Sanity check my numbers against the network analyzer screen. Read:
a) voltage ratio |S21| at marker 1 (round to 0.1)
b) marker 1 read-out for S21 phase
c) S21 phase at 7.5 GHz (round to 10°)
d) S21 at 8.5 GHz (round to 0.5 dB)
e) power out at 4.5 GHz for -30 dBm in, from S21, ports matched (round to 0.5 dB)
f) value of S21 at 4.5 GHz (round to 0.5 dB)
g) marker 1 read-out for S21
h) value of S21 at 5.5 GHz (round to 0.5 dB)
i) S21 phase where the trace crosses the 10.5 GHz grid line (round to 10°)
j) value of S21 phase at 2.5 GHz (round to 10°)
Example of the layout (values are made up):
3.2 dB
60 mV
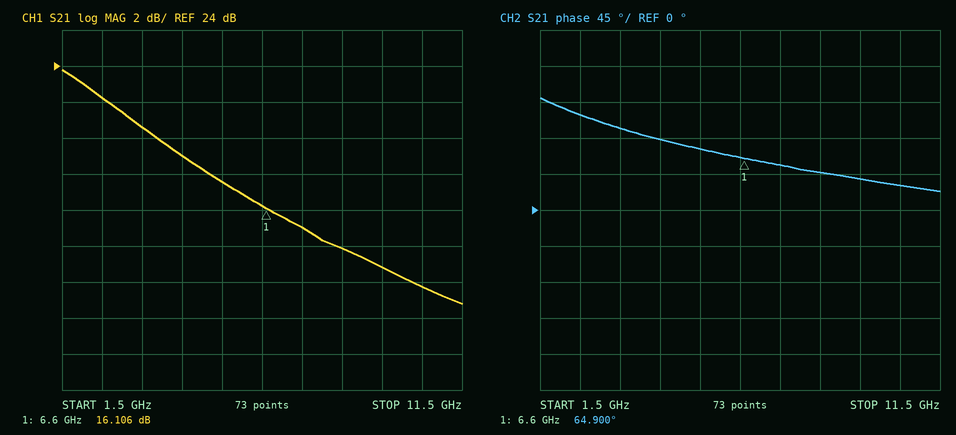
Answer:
6.4
64.900°
60°
14.0 dB
-11.0 dBm
19.0 dB
16.106 dB
17.5 dB
30°
120°
